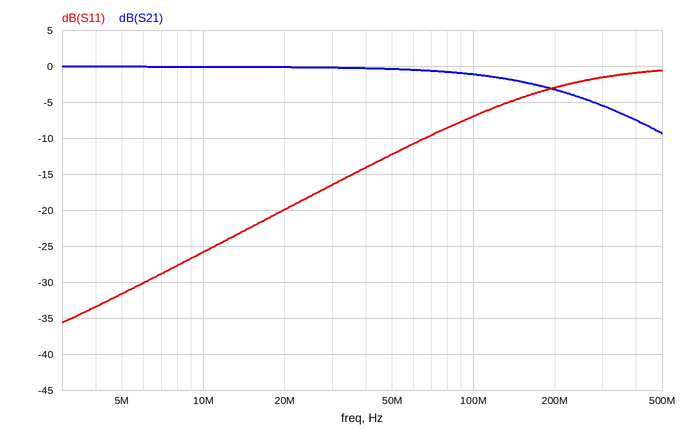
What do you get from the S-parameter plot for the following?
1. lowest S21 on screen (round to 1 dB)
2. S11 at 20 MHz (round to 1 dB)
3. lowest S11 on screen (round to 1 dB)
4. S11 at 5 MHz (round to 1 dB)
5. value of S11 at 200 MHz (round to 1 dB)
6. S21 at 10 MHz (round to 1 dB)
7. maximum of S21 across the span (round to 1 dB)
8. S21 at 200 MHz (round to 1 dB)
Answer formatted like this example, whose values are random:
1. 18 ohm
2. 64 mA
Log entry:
1. -9 dB
2. -20 dB
3. -36 dB
4. -32 dB
5. -3 dB
6. 0 dB
7. 0 dB
8. -3 dB
